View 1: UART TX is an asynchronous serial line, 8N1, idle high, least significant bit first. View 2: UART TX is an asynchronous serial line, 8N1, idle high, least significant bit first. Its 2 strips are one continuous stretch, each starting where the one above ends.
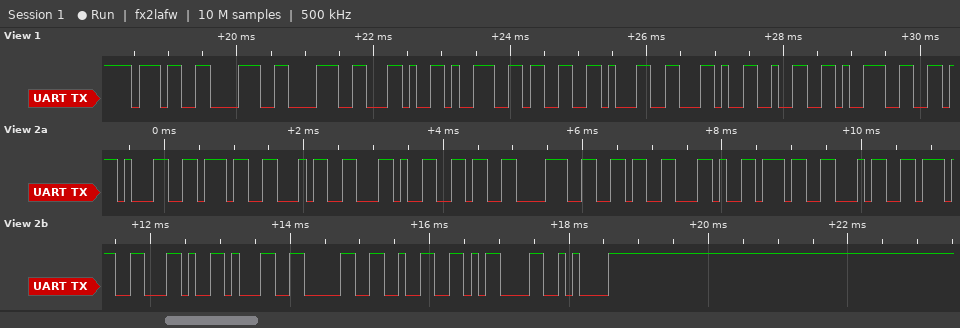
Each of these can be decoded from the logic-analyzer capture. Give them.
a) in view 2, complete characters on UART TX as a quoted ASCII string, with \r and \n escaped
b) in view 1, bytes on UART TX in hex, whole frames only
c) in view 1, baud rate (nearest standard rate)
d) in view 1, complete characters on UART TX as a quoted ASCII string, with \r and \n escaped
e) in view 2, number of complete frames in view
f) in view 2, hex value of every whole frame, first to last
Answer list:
"174,686,747,102\r\n"
37 38 38 2C 39 33 31 2C 32 39
9600 baud
"788,931,29"
17
31 37 34 2C 36 38 36 2C 37 34 37 2C 31 30 32 0D 0A
